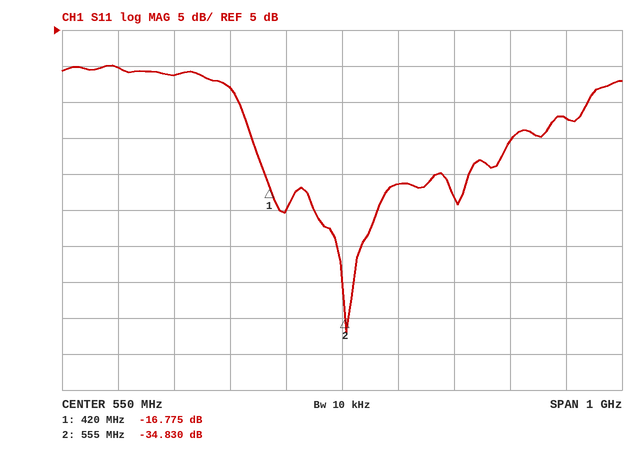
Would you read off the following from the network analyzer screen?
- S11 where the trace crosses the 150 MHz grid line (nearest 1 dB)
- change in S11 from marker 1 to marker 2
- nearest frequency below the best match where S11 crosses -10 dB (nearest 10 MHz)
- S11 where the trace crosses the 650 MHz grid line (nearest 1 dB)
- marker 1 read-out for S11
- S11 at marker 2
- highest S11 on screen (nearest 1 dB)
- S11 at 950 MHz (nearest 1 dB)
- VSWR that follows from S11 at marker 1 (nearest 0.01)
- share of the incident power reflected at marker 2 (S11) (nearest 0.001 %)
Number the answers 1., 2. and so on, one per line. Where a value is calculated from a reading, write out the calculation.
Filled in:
1. 0 dB
2. -34.83 − (-16.775) = -18.055 dB
3. 390 MHz
4. -16 dB
5. -16.775 dB
6. -34.830 dB
7. 0 dB
8. -7 dB
9. (1 + 0.1450)/(1 − 0.1450) ≈ 1.34
10. 10^(-34.83/10) ≈ 0.033 %
